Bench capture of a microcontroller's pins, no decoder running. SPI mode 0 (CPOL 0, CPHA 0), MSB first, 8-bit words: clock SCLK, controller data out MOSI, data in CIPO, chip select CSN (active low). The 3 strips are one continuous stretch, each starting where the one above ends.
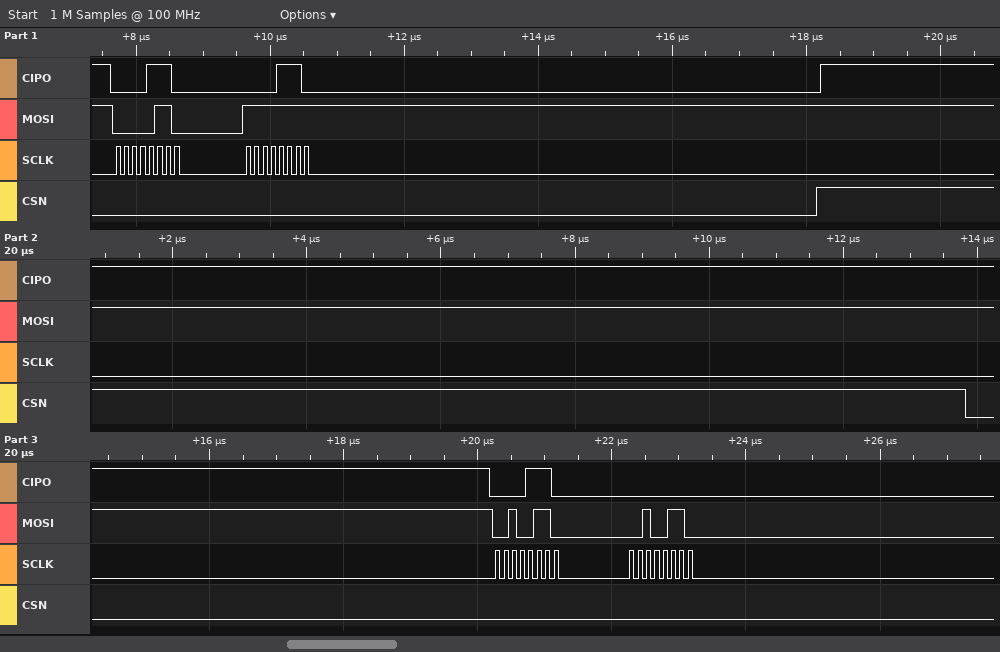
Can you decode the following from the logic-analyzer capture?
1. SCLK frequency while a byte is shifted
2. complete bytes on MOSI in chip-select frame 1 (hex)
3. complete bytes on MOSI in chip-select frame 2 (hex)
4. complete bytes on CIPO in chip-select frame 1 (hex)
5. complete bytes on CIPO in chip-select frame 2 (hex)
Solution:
8 MHz
0x06 0xFF
0x26 0x26
0x0E 0x0E
0x0E 0x00
